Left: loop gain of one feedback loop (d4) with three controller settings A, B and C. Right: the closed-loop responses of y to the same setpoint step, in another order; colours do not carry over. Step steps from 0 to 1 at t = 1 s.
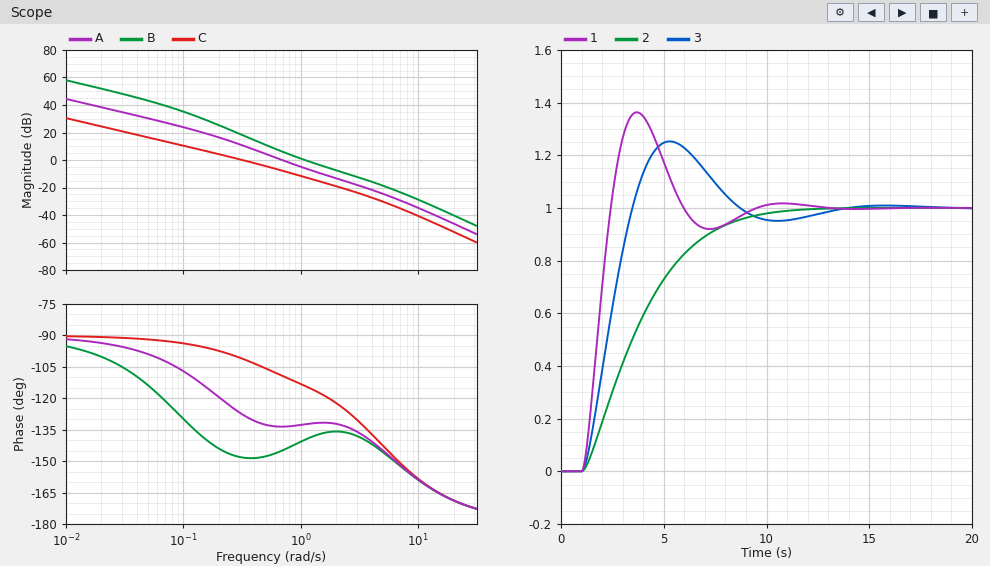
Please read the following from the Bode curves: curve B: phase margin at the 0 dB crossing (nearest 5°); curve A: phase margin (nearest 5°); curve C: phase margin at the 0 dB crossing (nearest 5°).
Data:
40°
45°
80°
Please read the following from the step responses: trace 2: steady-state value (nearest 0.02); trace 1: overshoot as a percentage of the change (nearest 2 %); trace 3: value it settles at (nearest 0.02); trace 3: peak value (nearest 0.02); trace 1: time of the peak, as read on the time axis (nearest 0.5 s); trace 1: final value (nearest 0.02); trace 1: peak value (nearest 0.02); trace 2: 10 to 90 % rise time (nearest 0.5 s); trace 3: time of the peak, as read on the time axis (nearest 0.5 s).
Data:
1.00
36 %
1.00
1.26
3.5 s
1.00
1.36
5.5 s
5.5 s
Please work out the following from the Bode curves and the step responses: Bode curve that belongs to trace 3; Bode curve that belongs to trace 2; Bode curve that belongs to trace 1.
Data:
A
C
B
